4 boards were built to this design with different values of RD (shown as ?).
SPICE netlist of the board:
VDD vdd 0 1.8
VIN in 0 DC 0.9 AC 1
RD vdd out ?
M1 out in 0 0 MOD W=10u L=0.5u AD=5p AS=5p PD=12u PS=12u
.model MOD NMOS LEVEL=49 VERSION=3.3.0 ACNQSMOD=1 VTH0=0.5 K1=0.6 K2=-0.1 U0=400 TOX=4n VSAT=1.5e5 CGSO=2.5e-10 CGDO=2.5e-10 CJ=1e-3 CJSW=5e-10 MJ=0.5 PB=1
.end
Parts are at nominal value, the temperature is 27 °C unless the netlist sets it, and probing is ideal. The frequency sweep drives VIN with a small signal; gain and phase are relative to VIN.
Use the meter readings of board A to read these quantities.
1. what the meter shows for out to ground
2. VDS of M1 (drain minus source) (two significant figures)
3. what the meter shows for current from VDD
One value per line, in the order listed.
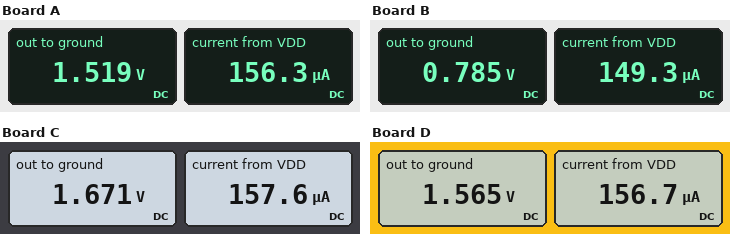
1.519 V
1.5 V
156.3 µA
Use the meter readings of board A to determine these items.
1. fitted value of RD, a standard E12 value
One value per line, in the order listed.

1.8 kΩ
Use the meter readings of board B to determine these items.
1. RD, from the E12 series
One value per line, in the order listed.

6.8 kΩ
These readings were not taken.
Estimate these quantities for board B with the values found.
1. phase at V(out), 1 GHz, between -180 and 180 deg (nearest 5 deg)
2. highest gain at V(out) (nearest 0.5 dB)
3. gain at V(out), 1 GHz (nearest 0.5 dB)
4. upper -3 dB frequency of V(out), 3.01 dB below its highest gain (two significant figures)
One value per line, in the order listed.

145 deg
15.0 dB
14.0 dB
2.1 GHz
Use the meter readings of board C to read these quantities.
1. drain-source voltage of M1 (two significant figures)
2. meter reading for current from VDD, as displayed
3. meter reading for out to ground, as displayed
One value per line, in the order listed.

1.7 V
157.6 µA
1.671 V
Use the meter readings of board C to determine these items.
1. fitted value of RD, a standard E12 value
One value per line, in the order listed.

820 Ω
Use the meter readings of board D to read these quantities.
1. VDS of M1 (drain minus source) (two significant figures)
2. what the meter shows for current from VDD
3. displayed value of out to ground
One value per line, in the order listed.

1.6 V
156.7 µA
1.565 V
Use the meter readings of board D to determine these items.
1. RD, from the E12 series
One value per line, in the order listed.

1.5 kΩ
